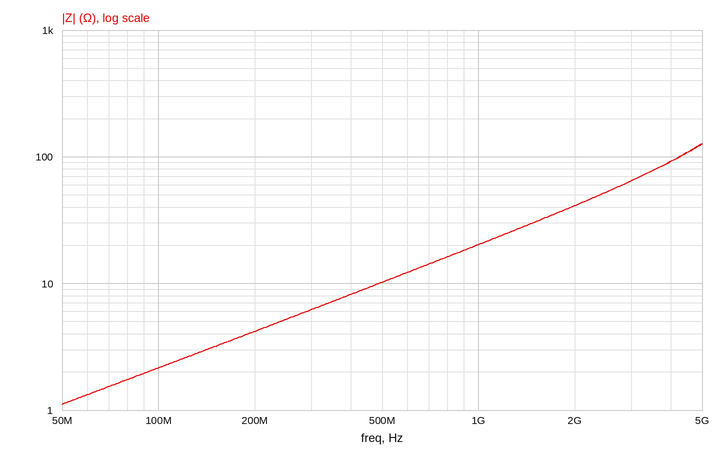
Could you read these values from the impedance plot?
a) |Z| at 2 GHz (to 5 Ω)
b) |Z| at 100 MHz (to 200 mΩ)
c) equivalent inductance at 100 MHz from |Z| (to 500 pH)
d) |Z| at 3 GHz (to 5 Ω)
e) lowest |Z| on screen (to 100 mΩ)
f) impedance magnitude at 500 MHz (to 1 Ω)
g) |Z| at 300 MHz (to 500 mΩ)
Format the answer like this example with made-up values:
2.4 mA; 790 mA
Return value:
40 Ω; 2.2 Ω; 3.5 nH; 65 Ω; 1.1 Ω; 10 Ω; 6.0 Ω
